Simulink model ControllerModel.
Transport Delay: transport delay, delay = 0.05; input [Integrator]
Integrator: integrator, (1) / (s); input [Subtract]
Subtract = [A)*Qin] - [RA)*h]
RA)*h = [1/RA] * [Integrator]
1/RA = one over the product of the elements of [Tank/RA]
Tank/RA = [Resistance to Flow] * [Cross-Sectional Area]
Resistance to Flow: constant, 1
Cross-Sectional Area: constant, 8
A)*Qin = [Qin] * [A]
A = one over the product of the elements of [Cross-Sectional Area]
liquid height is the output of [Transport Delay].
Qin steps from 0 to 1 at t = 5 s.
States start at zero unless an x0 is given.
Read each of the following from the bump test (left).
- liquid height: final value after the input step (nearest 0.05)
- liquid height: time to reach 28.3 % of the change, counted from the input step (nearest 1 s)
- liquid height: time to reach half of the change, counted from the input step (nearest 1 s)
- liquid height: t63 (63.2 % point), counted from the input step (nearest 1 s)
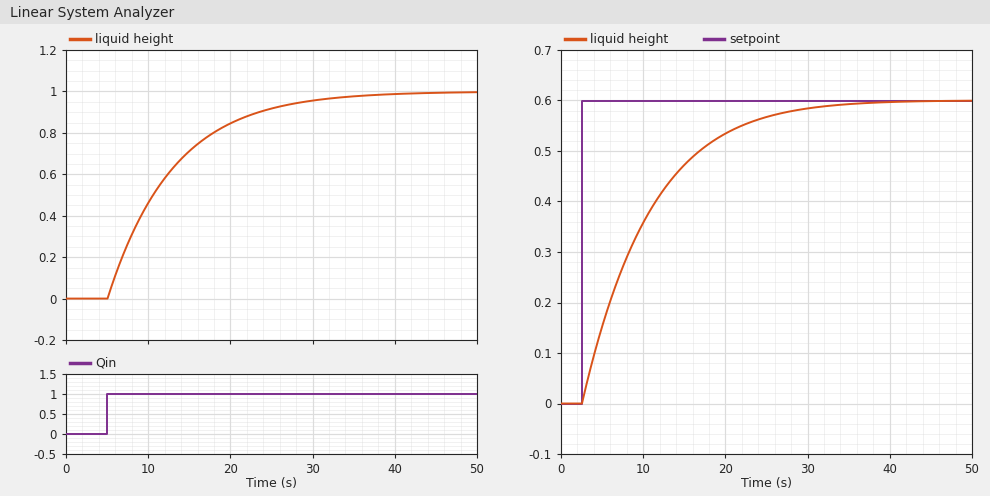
1.00
3 s
6 s
8 s
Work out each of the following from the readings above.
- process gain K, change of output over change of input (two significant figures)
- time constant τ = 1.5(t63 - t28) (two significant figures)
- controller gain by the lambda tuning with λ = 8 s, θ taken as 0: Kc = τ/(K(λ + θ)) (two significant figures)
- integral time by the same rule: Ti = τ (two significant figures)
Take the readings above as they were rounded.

1.0
7.5 s
0.94
7.5 s
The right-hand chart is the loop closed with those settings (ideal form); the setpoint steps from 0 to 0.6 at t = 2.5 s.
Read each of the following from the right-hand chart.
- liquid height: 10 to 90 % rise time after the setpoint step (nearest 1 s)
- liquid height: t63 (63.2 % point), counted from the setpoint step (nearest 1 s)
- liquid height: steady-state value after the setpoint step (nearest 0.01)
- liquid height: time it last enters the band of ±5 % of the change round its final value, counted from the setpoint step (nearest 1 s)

17 s
8 s
0.60
23 s
